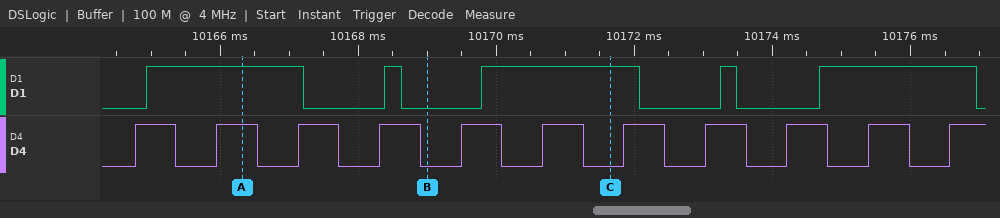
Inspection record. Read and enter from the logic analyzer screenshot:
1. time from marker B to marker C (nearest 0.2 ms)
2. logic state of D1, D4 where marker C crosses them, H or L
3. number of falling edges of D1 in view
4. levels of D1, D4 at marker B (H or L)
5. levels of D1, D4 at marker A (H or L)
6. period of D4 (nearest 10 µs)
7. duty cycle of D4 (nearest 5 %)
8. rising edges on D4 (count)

2.6 ms
D1=H, D4=L
5
D1=L, D4=L
D1=H, D4=H
1180 µs
50 %
11
